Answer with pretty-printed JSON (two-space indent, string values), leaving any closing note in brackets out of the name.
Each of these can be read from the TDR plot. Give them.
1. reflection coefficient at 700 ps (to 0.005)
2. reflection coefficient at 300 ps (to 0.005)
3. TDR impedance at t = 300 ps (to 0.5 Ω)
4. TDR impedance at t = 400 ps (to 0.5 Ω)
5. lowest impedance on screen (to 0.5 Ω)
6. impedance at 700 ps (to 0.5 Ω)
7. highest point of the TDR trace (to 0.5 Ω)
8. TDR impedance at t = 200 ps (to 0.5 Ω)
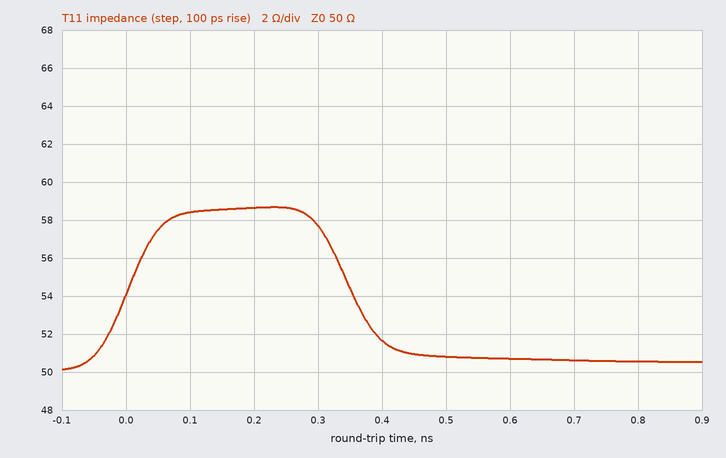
{
  "reflection coefficient at 700 ps": "+0.005",
  "reflection coefficient at 300 ps": "+0.070",
  "TDR impedance at t = 300 ps": "57.5 Ω",
  "TDR impedance at t = 400 ps": "51.5 Ω",
  "lowest impedance on screen": "50.0 Ω",
  "impedance at 700 ps": "50.5 Ω",
  "highest point of the TDR trace": "58.5 Ω",
  "TDR impedance at t = 200 ps": "58.5 Ω"
}
